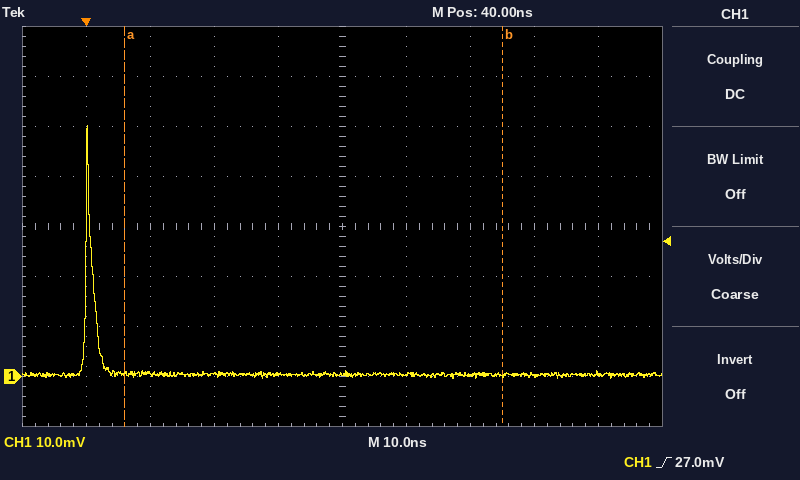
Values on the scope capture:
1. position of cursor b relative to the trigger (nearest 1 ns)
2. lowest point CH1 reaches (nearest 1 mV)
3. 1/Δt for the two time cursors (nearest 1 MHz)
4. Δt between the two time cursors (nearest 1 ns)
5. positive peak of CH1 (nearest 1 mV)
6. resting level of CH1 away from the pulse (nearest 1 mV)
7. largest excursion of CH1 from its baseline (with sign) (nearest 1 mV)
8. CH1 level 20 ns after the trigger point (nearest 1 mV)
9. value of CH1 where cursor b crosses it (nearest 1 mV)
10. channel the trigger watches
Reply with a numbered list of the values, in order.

1. +65 ns
2. 0 mV
3. 17 MHz
4. 59 ns
5. 50 mV
6. 0 mV
7. +50 mV
8. 1 mV
9. 0 mV
10. CH1
